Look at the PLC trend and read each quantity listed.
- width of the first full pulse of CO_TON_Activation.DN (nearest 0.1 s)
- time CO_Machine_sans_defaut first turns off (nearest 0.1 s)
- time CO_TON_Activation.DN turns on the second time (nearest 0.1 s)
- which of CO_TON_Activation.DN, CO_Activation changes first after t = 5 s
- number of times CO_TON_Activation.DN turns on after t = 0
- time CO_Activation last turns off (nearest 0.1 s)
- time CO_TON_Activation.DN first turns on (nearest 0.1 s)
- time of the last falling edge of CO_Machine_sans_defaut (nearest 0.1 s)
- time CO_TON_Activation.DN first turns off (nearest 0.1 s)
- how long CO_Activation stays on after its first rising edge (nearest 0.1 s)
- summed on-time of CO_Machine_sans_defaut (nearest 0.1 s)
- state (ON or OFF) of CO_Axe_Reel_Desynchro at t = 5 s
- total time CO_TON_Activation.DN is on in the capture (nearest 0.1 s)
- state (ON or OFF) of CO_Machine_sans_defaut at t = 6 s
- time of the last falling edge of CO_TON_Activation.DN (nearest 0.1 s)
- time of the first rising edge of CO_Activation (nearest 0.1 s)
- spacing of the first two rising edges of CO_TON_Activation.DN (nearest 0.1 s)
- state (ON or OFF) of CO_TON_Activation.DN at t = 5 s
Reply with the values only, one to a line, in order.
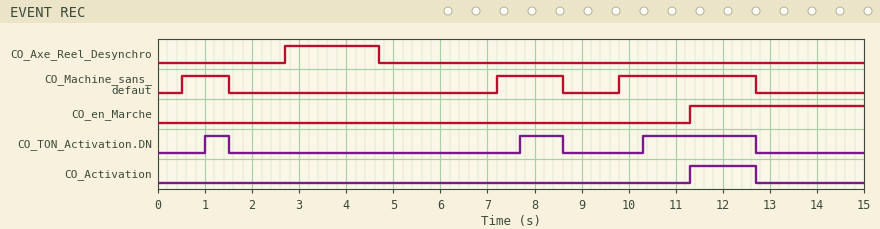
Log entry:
0.5 s
1.5 s
7.7 s
CO_TON_Activation.DN
3
12.7 s
1.0 s
12.7 s
1.5 s
1.4 s
5.3 s
OFF
3.8 s
OFF
12.7 s
11.3 s
6.7 s
OFF
